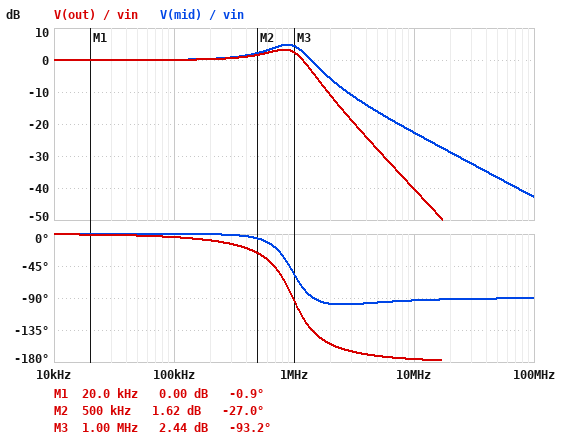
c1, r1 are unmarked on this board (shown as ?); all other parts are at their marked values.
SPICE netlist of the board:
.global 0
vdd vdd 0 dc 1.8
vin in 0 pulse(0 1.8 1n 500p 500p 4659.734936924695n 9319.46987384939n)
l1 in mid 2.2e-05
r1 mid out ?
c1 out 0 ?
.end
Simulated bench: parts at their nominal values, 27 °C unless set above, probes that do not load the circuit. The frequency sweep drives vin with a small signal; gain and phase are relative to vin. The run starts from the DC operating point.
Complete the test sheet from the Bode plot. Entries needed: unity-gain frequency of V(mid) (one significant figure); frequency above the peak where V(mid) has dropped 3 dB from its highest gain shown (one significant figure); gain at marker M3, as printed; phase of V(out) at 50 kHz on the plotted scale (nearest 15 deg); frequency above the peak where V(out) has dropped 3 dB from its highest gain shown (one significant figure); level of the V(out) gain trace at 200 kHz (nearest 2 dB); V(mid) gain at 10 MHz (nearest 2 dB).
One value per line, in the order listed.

1 MHz
1 MHz
2.44 dB
0 deg
1 MHz
0 dB
-22 dB
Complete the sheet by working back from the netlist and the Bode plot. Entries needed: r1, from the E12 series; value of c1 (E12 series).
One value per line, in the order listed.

100 Ω
1.2 nF
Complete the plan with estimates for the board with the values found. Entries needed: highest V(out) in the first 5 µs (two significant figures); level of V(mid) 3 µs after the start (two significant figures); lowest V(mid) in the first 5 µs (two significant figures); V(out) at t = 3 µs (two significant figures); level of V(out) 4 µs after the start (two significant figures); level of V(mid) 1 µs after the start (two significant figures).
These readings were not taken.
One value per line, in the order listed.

2.3 V
1.8 V
-610 mV
1.8 V
1.8 V
1.6 V
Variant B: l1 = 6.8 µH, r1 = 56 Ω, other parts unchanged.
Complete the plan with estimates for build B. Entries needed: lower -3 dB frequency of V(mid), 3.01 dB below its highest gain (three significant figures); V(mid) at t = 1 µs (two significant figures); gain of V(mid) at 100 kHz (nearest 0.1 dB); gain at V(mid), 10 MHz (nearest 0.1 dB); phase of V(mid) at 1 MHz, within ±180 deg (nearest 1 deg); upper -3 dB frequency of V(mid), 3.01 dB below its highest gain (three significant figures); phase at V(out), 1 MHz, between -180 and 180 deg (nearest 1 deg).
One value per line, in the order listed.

799 kHz
1.8 V
0 dB
-17.2 dB
-9 deg
2.24 MHz
-32 deg
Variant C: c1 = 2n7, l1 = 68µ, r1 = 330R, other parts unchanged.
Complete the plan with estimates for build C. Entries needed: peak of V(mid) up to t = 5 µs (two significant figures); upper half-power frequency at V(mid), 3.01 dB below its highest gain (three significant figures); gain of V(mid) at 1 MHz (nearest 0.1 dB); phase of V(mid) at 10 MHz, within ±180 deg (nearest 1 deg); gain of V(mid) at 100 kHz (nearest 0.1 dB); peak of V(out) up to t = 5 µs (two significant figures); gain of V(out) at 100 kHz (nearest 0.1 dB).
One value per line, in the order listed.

2.0 V
778 kHz
-3.4 dB
-87 deg
0.5 dB
1.8 V
-0.7 dB
